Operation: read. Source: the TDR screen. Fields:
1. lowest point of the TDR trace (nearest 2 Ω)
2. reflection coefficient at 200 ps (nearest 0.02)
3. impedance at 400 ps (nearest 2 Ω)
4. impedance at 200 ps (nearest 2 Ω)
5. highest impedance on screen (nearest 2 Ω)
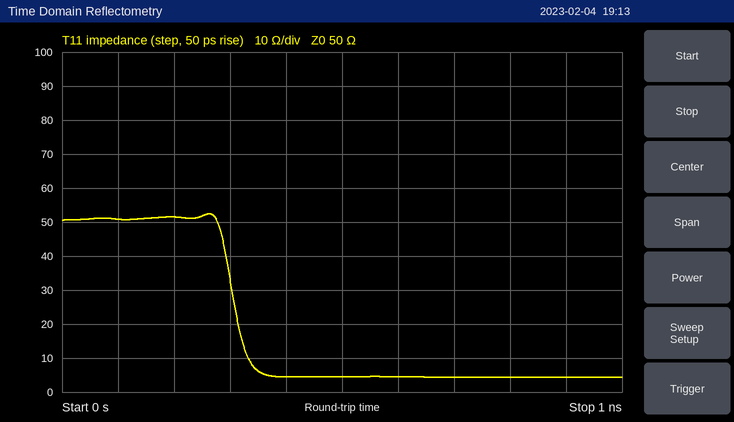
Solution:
4 Ω
+0.02
4 Ω
52 Ω
52 Ω
